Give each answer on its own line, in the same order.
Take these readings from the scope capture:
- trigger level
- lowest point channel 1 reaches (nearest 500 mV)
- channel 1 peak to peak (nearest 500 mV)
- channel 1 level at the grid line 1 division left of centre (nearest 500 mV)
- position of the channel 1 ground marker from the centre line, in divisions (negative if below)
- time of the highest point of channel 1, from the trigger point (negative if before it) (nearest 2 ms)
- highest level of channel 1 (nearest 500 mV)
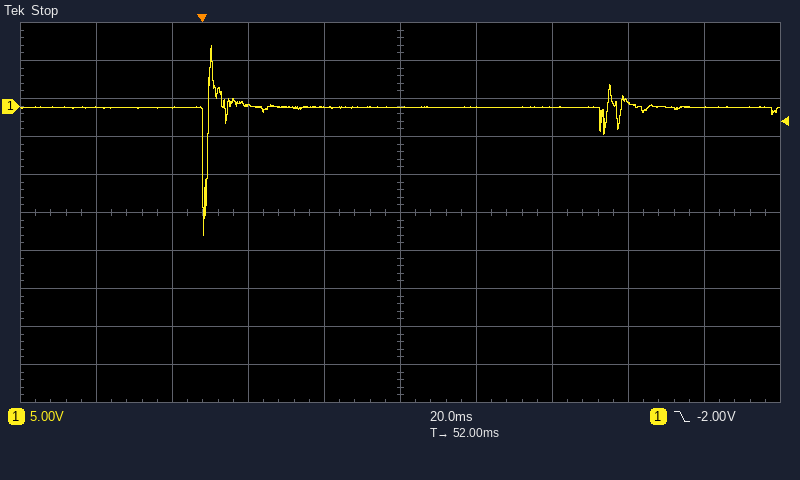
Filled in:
-2.00 V
-17.0 V
25.0 V
0.0 V
+2.8 div
+2 ms
8.0 V
